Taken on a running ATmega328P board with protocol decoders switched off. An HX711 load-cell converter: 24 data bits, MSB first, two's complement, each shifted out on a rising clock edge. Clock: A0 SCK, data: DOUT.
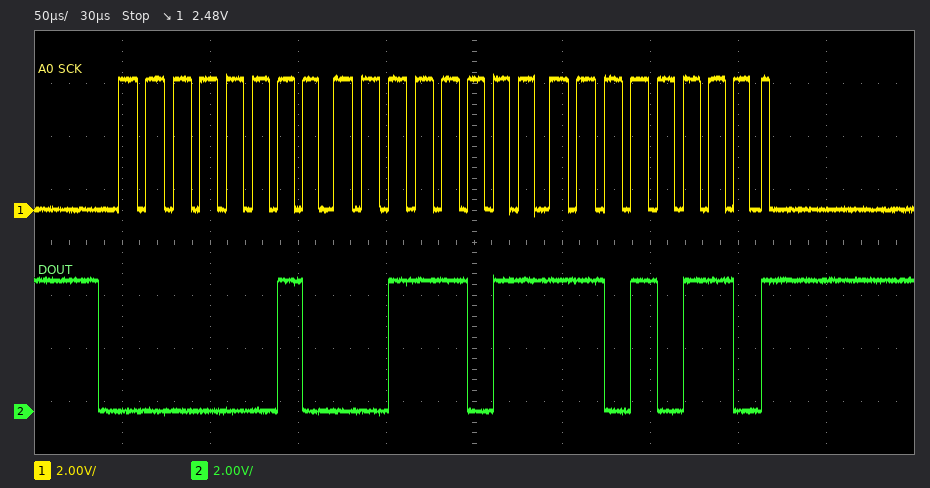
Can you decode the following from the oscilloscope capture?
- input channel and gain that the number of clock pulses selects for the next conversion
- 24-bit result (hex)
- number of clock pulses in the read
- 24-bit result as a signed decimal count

channel A, gain 128
0x023BD6
25
146390
